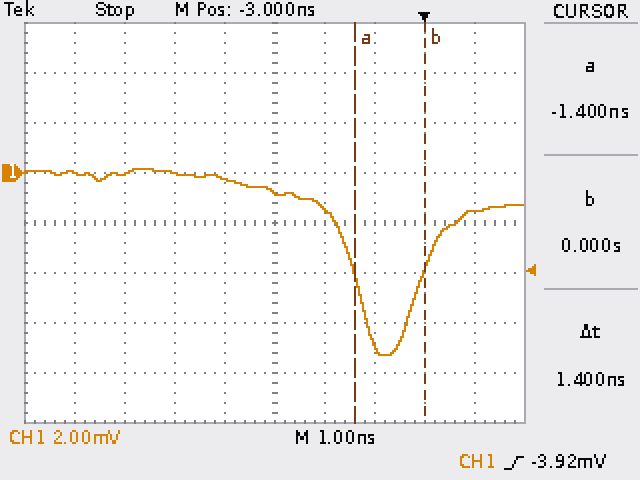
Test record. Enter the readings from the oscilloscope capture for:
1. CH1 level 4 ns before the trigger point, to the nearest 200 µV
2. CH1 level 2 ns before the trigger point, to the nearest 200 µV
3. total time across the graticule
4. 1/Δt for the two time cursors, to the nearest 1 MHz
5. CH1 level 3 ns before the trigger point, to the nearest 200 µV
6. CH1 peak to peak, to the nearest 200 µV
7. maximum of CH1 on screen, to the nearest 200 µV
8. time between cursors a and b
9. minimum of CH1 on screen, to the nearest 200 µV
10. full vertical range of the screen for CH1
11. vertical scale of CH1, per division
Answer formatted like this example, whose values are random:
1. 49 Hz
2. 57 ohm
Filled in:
1. -200 µV
2. -1.4 mV
3. 10 ns
4. 714 MHz
5. -800 µV
6. 7.4 mV
7. 200 µV
8. 1.4 ns
9. -7.2 mV
10. 16 mV
11. 2 mV
